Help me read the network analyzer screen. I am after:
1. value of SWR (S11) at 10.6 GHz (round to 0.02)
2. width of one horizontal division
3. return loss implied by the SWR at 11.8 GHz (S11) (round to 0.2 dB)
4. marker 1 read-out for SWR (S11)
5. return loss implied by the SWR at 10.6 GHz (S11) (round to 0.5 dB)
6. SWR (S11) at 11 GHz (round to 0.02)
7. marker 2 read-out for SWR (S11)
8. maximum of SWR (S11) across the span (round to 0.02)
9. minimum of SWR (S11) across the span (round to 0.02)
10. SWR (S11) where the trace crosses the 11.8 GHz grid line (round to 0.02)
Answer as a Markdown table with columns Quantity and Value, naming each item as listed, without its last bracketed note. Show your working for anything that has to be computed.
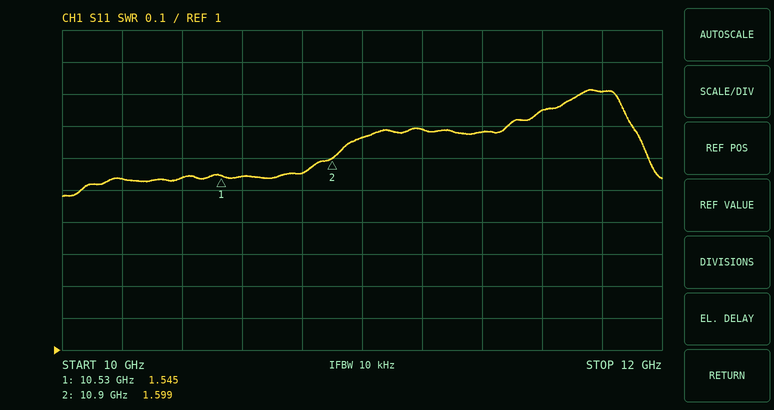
| Quantity | Value |
|---|---|
| value of SWR (S11) at 10.6 GHz | 1.54 |
| width of one horizontal division | 200 MHz |
| return loss implied by the SWR at 11.8 GHz (S11) | −20 log10((1.8 − 1)/(1.8 + 1)) ≈ 10.9 dB, so 10.8 dB to the nearest 0.2 dB |
| marker 1 read-out for SWR | 1.545 |
| return loss implied by the SWR at 10.6 GHz (S11) | −20 log10((1.54 − 1)/(1.54 + 1)) ≈ 13.4 dB, so 13.5 dB to the nearest 0.5 dB |
| SWR (S11) at 11 GHz | 1.66 |
| marker 2 read-out for SWR | 1.599 |
| maximum of SWR (S11) across the span | 1.82 |
| minimum of SWR (S11) across the span | 1.48 |
| SWR (S11) where the trace crosses the 11.8 GHz grid line | 1.80 |
